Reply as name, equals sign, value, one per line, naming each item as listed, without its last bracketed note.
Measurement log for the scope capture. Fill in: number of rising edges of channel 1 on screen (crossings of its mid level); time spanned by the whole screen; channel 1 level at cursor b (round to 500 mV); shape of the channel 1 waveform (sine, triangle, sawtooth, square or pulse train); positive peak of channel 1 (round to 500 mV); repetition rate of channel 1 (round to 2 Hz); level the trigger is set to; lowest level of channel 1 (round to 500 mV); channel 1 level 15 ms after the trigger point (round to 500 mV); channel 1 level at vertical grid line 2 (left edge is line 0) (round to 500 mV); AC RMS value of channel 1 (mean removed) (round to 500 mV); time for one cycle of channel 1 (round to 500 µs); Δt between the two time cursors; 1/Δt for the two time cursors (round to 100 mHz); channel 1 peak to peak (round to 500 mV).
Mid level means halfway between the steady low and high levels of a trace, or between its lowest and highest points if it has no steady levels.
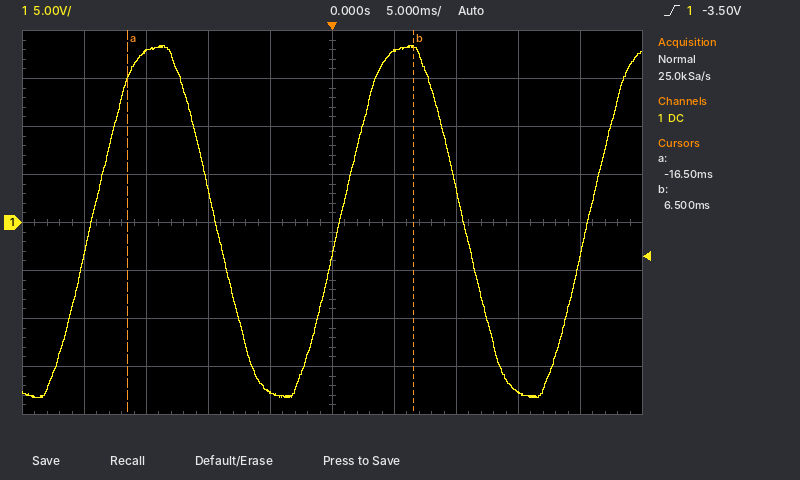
number of rising edges of channel 1 on screen = 3
time spanned by the whole screen = 50 ms
channel 1 level at cursor b = 18.0 V
shape of the channel 1 waveform = sine
positive peak of channel 1 = 18.5 V
repetition rate of channel 1 = 50 Hz
level the trigger is set to = -3.50 V
lowest level of channel 1 = -18.0 V
channel 1 level 15 ms after the trigger point = -17.5 V
channel 1 level at vertical grid line 2 (left edge is line 0) = 18.0 V
AC RMS value of channel 1 (mean removed) = 13.0 V
time for one cycle of channel 1 = 20.0 ms
Δt between the two time cursors = 23.0 ms
1/Δt for the two time cursors = 43.5 Hz
channel 1 peak to peak = 36.5 V
